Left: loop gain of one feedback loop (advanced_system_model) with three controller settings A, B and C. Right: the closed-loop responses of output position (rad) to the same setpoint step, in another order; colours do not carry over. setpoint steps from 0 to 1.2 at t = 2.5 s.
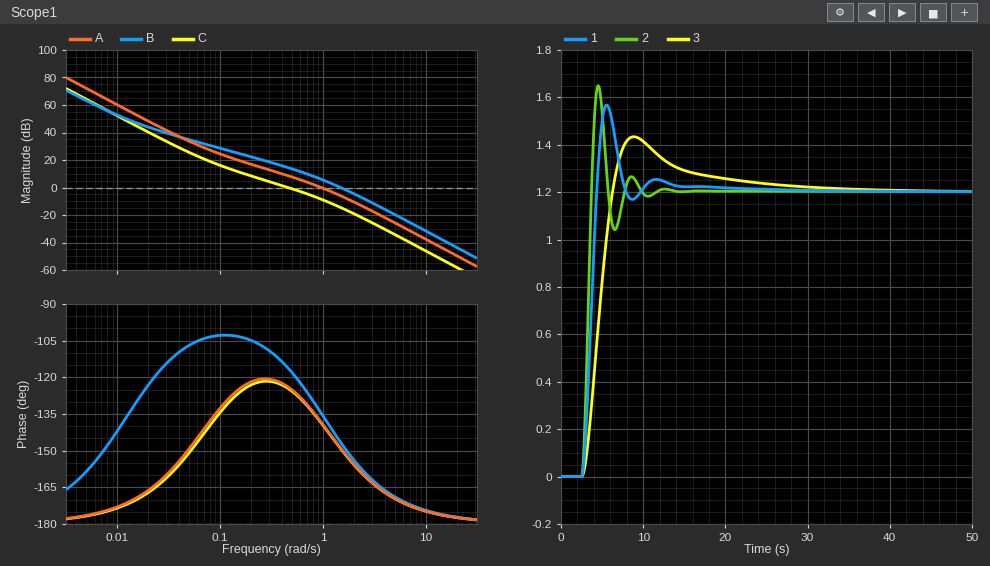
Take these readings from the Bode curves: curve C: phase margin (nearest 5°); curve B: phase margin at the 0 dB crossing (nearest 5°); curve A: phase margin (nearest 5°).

55°
35°
40°
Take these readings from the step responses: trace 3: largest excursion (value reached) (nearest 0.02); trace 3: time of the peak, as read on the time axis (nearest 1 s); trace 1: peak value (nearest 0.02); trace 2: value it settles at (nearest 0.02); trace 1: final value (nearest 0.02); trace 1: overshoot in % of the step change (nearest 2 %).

1.44
9 s
1.56
1.20
1.20
30 %
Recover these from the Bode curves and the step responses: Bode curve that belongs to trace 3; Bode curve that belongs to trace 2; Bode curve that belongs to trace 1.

C
B
A
